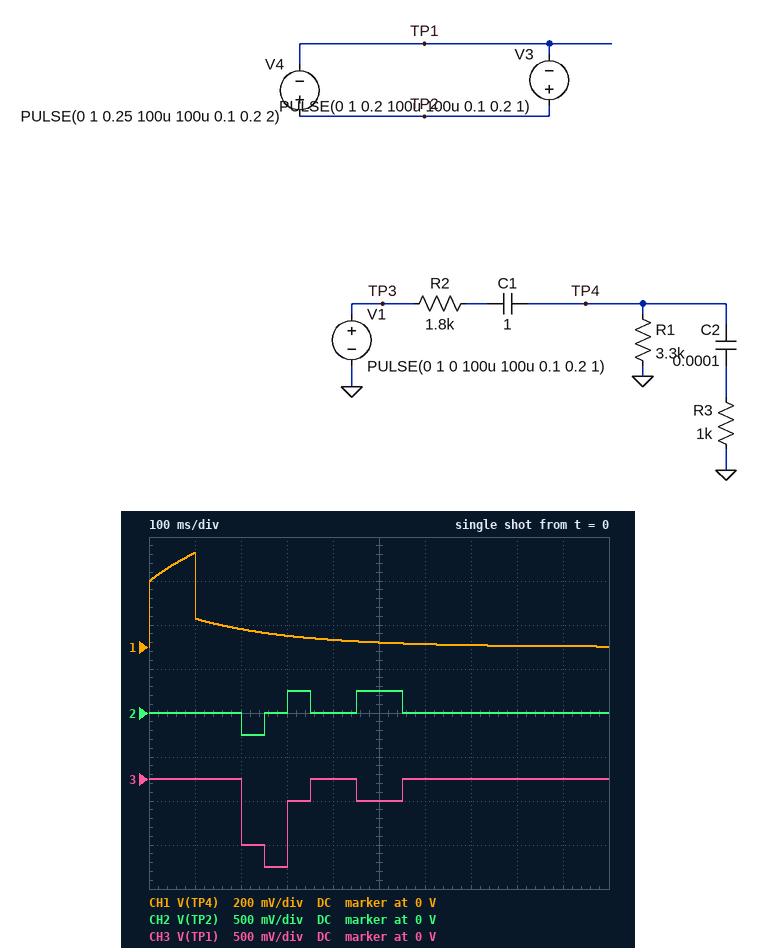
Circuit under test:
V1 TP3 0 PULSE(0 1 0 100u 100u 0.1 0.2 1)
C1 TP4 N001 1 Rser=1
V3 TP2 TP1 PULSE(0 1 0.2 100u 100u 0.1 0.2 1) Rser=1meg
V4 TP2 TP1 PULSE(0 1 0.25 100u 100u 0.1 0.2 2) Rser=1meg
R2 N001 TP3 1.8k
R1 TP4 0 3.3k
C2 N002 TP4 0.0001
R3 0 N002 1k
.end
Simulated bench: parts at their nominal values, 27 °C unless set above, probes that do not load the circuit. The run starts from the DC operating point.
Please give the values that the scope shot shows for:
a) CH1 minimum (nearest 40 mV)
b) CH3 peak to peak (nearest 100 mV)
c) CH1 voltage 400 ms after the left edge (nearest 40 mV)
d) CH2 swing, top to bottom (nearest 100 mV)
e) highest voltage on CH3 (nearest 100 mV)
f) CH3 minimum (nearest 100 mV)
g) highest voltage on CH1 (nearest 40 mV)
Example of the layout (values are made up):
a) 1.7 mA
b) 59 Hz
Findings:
a) 0 V
b) 1.0 V
c) 40 mV
d) 500 mV
e) 0 V
f) -1.0 V
g) 440 mV
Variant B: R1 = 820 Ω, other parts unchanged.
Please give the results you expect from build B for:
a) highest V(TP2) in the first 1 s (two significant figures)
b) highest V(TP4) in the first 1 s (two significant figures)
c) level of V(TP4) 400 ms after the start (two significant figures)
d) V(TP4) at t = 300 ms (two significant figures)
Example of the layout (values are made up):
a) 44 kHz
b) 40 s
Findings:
a) 250 mV
b) 250 mV
c) 7.8 mV
d) 15 mV
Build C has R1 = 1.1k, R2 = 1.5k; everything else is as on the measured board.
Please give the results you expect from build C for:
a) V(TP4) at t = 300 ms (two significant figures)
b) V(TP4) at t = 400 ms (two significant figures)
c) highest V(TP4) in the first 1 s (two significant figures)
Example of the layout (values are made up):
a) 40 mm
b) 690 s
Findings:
a) 22 mV
b) 12 mV
c) 330 mV
